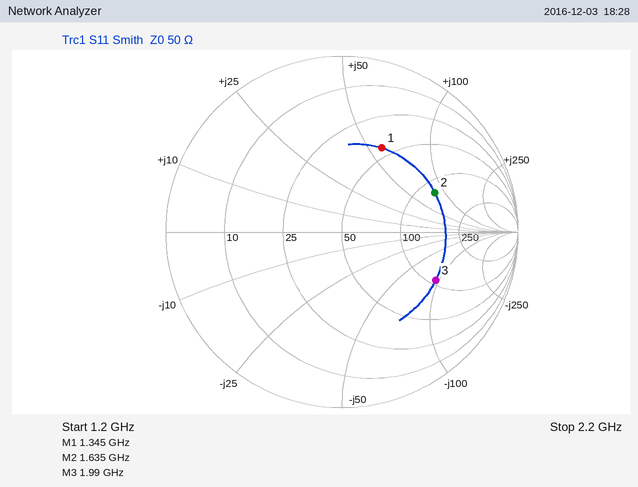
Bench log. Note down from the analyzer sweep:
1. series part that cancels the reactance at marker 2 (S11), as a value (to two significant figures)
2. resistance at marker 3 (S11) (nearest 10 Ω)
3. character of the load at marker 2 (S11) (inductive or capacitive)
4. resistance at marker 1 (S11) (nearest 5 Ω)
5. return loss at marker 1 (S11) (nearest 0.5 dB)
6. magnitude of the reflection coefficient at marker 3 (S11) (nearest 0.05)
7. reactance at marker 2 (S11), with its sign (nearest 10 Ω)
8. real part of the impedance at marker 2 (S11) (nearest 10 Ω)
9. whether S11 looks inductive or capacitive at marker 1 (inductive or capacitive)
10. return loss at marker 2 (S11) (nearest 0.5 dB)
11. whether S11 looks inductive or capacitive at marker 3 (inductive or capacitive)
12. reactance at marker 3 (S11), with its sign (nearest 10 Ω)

1.2 pF
110 Ω
inductive
45 Ω
5.5 dB
0.60
+80 Ω
120 Ω
inductive
5.0 dB
capacitive
-90 Ω
